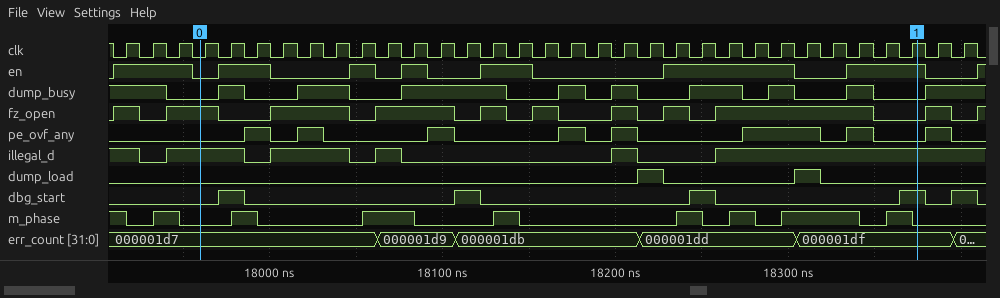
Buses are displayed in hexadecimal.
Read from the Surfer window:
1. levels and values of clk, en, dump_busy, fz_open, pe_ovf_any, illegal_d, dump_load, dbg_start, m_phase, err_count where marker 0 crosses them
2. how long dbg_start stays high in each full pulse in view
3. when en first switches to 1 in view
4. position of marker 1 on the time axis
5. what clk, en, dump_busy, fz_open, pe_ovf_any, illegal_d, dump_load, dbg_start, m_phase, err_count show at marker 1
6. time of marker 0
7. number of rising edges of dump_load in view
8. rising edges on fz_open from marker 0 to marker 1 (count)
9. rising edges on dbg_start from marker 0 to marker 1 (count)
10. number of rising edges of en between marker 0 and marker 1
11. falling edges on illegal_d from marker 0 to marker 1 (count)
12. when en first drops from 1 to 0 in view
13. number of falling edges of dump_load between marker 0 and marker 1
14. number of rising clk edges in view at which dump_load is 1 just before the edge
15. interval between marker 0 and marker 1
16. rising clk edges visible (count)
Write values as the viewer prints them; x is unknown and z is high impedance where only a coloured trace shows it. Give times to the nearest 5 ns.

clk=0, en=0, dump_busy=0, fz_open=1, pe_ovf_any=0, illegal_d=1, dump_load=0, dbg_start=0, m_phase=0, err_count=000001d7
15 ns, 15 ns, 15 ns, 15 ns, 15 ns
17910 ns
18375 ns
clk=1, en=1, dump_busy=0, fz_open=0, pe_ovf_any=0, illegal_d=1, dump_load=0, dbg_start=1, m_phase=0, err_count=000001df
17960 ns
2
7
4
6
4
17955 ns
2
2
415 ns
33
